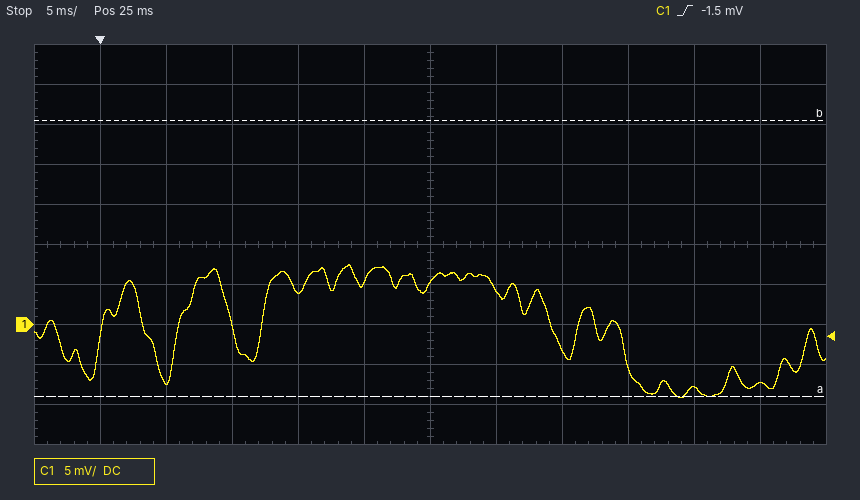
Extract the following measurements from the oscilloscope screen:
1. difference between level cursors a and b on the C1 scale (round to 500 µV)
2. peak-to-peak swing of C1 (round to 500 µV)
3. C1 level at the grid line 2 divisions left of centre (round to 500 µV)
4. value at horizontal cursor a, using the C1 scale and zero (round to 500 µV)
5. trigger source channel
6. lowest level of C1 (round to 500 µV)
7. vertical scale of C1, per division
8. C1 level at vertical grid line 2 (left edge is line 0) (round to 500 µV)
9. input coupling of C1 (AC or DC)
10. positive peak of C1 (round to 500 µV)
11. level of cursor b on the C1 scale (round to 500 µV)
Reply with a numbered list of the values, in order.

1. 34.5 mV
2. 16.5 mV
3. 4.0 mV
4. -9.0 mV
5. C1
6. -9.0 mV
7. 5 mV
8. -7.0 mV
9. DC
10. 7.5 mV
11. 25.5 mV
